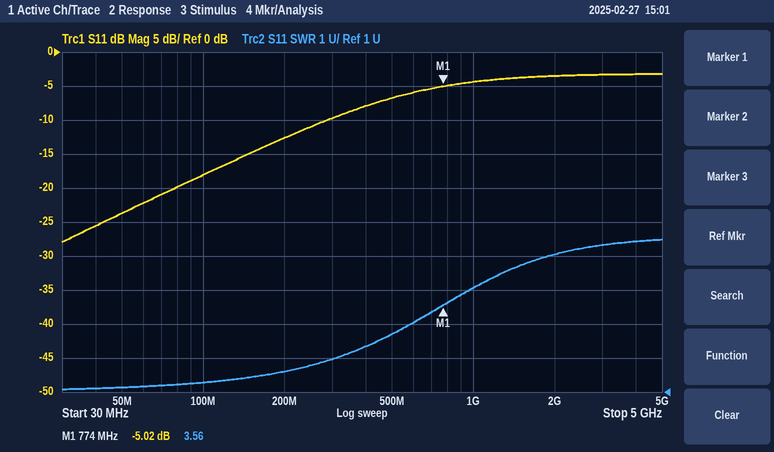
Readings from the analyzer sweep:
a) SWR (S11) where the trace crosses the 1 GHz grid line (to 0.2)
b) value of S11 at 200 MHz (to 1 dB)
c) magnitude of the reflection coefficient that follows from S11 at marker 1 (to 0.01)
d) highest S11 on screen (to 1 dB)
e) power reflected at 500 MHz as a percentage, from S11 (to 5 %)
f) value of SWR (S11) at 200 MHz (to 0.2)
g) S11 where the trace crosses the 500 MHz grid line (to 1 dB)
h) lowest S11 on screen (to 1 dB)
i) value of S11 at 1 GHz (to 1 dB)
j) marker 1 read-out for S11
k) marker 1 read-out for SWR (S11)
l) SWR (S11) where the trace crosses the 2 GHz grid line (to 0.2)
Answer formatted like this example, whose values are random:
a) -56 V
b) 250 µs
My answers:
a) 4.0
b) -13 dB
c) 0.56
d) -3 dB
e) 20 %
f) 1.6
g) -7 dB
h) -28 dB
i) -4 dB
j) -5.02 dB
k) 3.56
l) 5.0
